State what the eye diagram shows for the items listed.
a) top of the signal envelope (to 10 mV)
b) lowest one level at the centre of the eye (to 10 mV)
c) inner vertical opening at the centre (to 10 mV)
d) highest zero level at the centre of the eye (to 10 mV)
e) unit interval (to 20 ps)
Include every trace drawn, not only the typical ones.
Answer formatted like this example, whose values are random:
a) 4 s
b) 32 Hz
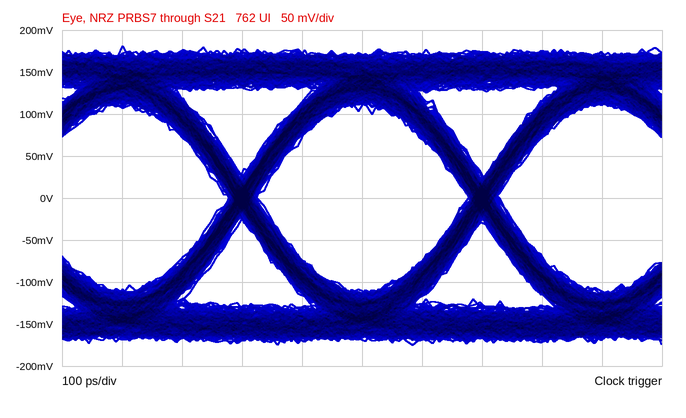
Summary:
a) 180 mV
b) 110 mV
c) 220 mV
d) -110 mV
e) 400 ps
